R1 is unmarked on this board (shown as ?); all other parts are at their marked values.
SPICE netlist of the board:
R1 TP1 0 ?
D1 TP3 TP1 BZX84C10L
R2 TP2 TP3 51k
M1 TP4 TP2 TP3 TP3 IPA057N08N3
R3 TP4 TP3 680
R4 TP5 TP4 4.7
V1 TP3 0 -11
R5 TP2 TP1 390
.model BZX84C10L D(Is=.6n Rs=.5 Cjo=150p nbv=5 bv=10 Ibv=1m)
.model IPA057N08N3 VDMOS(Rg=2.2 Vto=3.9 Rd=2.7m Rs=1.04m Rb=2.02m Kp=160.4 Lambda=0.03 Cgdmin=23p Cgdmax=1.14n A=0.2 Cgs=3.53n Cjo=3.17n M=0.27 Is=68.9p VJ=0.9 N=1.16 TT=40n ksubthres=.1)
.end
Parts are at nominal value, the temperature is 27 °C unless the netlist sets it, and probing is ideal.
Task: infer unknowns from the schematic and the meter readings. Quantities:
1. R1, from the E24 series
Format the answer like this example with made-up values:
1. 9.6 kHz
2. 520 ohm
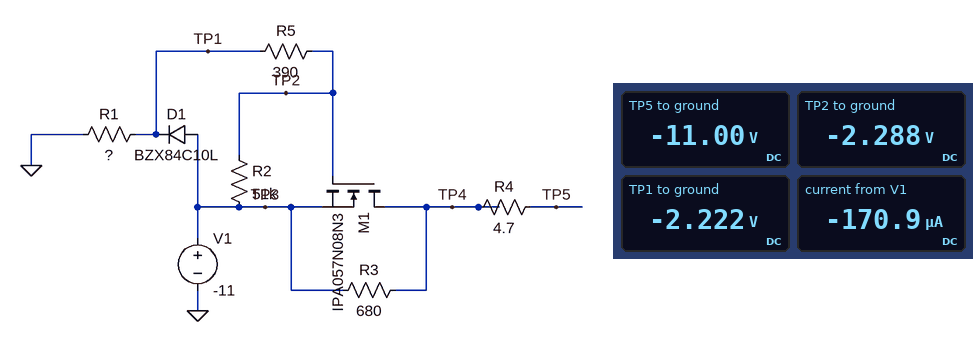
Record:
1. 13 kΩ
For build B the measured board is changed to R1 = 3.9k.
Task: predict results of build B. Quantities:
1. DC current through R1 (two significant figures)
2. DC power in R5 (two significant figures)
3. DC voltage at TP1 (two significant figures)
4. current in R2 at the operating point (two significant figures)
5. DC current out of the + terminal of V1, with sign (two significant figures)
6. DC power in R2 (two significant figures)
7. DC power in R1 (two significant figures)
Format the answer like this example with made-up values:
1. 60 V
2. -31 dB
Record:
1. 320 µA
2. 14 µW
3. -1.3 V
4. 190 µA
5. -320 µA
6. 1.8 mW
7. 410 µW
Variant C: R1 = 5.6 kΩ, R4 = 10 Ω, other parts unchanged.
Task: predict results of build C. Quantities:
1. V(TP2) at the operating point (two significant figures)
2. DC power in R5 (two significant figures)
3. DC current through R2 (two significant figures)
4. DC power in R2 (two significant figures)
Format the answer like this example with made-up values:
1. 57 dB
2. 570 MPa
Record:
1. -1.4 V
2. 14 µW
3. 190 µA
4. 1.8 mW
